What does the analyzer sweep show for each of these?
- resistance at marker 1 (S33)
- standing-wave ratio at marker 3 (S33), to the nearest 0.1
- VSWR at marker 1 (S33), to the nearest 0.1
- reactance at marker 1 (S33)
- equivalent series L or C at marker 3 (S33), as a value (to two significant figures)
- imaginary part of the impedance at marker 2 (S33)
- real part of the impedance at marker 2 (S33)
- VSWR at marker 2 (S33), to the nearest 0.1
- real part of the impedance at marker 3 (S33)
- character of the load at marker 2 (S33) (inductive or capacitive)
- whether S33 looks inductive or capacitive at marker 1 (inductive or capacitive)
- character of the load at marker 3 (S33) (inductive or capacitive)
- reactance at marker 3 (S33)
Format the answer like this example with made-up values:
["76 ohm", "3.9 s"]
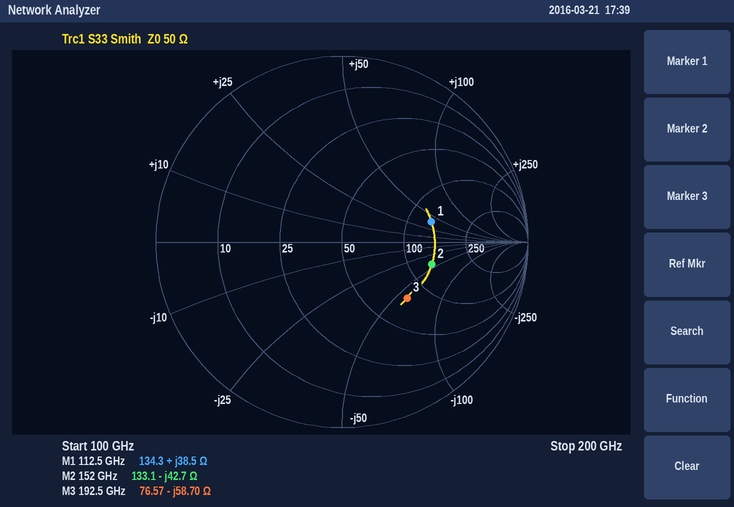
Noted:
["134.3 Ω", "2.7", "2.9", "+38.5 Ω", "14 fF", "-42.7 Ω", "133.1 Ω", "3.0", "76.57 Ω", "capacitive", "inductive", "capacitive", "-58.70 Ω"]
